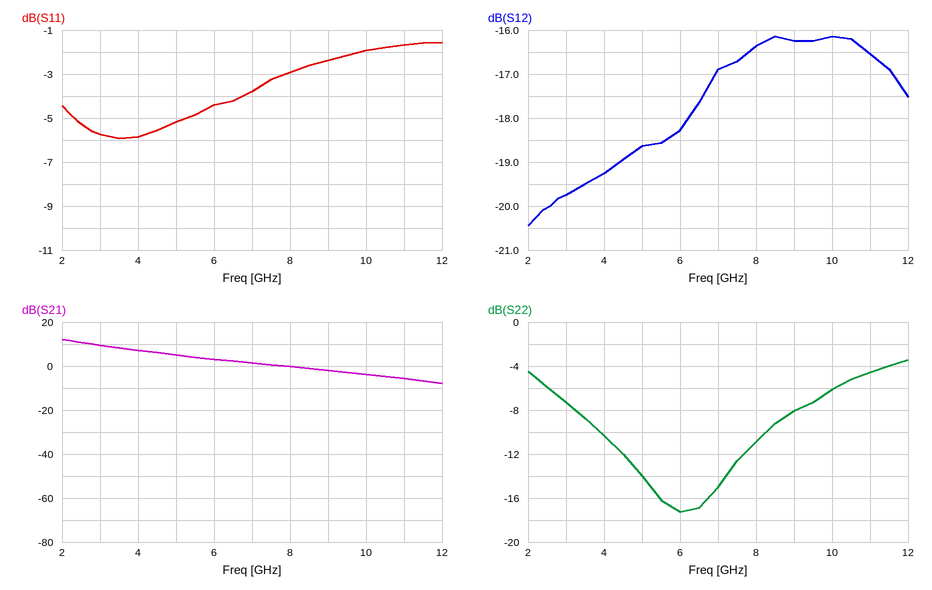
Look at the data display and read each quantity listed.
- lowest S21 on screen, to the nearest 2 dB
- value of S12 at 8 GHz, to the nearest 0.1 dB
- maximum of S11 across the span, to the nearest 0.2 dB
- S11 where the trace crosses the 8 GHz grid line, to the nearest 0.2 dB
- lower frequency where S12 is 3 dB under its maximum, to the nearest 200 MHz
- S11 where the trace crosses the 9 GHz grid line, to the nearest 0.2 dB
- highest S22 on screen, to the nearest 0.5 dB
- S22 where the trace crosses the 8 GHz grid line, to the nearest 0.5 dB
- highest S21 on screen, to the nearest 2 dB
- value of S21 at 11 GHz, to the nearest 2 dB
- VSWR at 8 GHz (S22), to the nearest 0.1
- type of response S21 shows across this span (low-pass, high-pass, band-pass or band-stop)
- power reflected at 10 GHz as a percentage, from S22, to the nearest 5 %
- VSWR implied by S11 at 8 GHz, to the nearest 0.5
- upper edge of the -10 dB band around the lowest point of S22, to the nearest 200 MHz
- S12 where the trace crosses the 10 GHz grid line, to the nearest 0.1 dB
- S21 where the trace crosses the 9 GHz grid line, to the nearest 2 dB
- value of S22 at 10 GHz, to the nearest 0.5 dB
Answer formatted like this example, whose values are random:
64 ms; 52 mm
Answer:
-8 dB; -16.4 dB; -1.6 dB; -3.0 dB; 4.2 GHz; -2.4 dB; -3.5 dB; -11.0 dB; 12 dB; -6 dB; 1.8; low-pass; 25 %; 6.0; 8.2 GHz; -16.1 dB; -2 dB; -6.0 dB
